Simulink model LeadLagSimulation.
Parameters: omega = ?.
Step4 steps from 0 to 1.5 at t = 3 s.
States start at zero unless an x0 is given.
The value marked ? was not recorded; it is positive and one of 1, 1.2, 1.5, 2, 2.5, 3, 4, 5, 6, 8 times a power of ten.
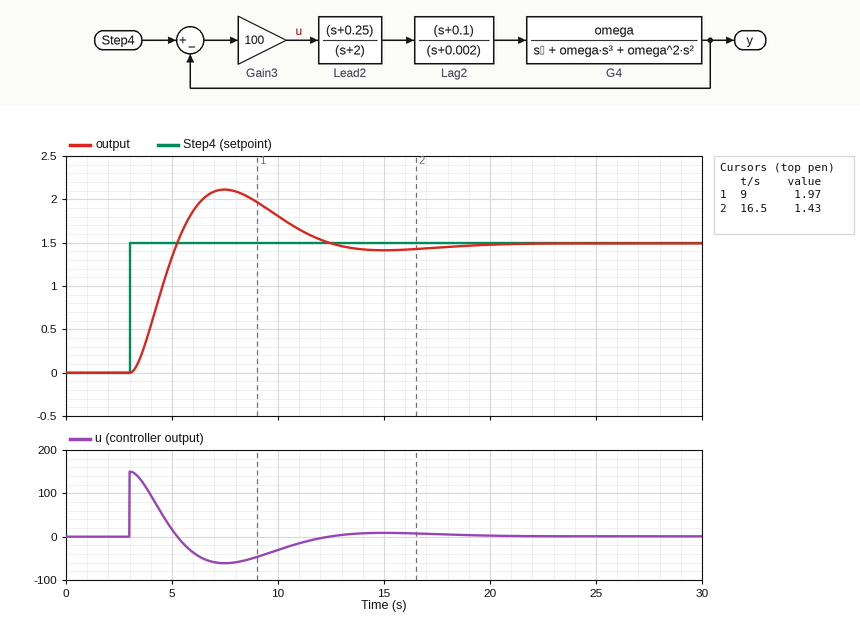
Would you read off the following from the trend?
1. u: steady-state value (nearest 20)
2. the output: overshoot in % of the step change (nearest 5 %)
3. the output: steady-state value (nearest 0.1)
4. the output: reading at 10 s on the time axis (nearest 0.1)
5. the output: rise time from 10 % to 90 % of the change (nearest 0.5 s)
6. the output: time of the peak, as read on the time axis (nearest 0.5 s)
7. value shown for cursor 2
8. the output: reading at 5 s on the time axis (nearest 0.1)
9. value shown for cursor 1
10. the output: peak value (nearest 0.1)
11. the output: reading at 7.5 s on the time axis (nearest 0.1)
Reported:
0
40 %
1.5
1.8
1.5 s
7.5 s
1.43
1.3
1.97
2.1
2.1
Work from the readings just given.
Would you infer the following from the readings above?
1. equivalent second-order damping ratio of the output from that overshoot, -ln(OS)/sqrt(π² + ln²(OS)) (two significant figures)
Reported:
0.28
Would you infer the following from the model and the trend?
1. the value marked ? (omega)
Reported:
80
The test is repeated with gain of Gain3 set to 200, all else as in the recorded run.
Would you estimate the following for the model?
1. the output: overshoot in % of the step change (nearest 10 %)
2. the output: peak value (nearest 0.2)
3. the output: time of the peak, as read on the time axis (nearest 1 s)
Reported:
40 %
2.0
6 s
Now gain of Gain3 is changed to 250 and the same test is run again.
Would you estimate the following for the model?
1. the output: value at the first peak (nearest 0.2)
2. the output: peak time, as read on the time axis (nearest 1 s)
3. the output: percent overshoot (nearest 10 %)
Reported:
2.0
5 s
40 %
